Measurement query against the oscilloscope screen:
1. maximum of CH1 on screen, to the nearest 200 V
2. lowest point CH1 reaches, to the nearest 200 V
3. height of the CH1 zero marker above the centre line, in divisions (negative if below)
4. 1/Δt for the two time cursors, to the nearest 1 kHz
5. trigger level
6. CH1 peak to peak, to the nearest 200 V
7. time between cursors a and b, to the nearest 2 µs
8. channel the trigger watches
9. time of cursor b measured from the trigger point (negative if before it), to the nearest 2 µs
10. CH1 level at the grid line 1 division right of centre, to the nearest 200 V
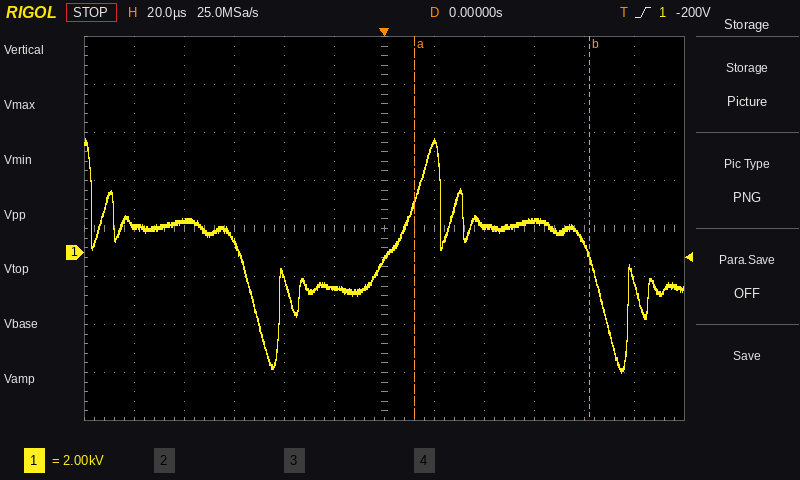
4.8 kV
-5.0 kV
-0.5 div
14 kHz
-200 V
9.8 kV
70 µs
CH1
+82 µs
4.6 kV
